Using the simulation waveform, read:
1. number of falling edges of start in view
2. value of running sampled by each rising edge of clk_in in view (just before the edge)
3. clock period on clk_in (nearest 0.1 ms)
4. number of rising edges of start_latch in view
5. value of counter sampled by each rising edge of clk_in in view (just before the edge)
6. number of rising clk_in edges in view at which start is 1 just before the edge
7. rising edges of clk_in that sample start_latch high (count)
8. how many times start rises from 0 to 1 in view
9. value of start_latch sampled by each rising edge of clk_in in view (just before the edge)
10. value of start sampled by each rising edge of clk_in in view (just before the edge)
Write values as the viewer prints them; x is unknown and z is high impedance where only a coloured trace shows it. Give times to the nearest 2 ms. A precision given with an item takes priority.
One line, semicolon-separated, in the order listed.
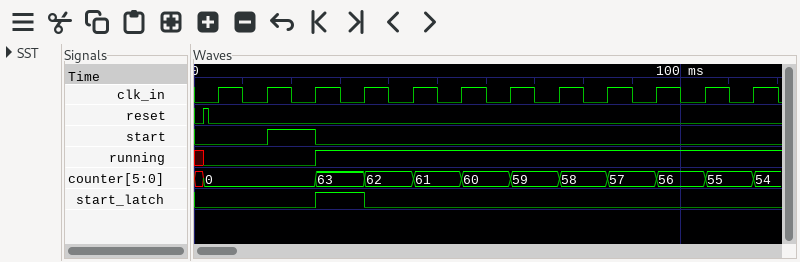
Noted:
1; 0 0 0 1 1 1 1 1 1 1 1 1; 10 ms; 1; 0, 0, 0, 63, 62, 61, 60, 59, 58, 57, 56, 55; 1; 1; 1; 0 0 0 1 0 0 0 0 0 0 0 0; 0 0 1 0 0 0 0 0 0 0 0 0
